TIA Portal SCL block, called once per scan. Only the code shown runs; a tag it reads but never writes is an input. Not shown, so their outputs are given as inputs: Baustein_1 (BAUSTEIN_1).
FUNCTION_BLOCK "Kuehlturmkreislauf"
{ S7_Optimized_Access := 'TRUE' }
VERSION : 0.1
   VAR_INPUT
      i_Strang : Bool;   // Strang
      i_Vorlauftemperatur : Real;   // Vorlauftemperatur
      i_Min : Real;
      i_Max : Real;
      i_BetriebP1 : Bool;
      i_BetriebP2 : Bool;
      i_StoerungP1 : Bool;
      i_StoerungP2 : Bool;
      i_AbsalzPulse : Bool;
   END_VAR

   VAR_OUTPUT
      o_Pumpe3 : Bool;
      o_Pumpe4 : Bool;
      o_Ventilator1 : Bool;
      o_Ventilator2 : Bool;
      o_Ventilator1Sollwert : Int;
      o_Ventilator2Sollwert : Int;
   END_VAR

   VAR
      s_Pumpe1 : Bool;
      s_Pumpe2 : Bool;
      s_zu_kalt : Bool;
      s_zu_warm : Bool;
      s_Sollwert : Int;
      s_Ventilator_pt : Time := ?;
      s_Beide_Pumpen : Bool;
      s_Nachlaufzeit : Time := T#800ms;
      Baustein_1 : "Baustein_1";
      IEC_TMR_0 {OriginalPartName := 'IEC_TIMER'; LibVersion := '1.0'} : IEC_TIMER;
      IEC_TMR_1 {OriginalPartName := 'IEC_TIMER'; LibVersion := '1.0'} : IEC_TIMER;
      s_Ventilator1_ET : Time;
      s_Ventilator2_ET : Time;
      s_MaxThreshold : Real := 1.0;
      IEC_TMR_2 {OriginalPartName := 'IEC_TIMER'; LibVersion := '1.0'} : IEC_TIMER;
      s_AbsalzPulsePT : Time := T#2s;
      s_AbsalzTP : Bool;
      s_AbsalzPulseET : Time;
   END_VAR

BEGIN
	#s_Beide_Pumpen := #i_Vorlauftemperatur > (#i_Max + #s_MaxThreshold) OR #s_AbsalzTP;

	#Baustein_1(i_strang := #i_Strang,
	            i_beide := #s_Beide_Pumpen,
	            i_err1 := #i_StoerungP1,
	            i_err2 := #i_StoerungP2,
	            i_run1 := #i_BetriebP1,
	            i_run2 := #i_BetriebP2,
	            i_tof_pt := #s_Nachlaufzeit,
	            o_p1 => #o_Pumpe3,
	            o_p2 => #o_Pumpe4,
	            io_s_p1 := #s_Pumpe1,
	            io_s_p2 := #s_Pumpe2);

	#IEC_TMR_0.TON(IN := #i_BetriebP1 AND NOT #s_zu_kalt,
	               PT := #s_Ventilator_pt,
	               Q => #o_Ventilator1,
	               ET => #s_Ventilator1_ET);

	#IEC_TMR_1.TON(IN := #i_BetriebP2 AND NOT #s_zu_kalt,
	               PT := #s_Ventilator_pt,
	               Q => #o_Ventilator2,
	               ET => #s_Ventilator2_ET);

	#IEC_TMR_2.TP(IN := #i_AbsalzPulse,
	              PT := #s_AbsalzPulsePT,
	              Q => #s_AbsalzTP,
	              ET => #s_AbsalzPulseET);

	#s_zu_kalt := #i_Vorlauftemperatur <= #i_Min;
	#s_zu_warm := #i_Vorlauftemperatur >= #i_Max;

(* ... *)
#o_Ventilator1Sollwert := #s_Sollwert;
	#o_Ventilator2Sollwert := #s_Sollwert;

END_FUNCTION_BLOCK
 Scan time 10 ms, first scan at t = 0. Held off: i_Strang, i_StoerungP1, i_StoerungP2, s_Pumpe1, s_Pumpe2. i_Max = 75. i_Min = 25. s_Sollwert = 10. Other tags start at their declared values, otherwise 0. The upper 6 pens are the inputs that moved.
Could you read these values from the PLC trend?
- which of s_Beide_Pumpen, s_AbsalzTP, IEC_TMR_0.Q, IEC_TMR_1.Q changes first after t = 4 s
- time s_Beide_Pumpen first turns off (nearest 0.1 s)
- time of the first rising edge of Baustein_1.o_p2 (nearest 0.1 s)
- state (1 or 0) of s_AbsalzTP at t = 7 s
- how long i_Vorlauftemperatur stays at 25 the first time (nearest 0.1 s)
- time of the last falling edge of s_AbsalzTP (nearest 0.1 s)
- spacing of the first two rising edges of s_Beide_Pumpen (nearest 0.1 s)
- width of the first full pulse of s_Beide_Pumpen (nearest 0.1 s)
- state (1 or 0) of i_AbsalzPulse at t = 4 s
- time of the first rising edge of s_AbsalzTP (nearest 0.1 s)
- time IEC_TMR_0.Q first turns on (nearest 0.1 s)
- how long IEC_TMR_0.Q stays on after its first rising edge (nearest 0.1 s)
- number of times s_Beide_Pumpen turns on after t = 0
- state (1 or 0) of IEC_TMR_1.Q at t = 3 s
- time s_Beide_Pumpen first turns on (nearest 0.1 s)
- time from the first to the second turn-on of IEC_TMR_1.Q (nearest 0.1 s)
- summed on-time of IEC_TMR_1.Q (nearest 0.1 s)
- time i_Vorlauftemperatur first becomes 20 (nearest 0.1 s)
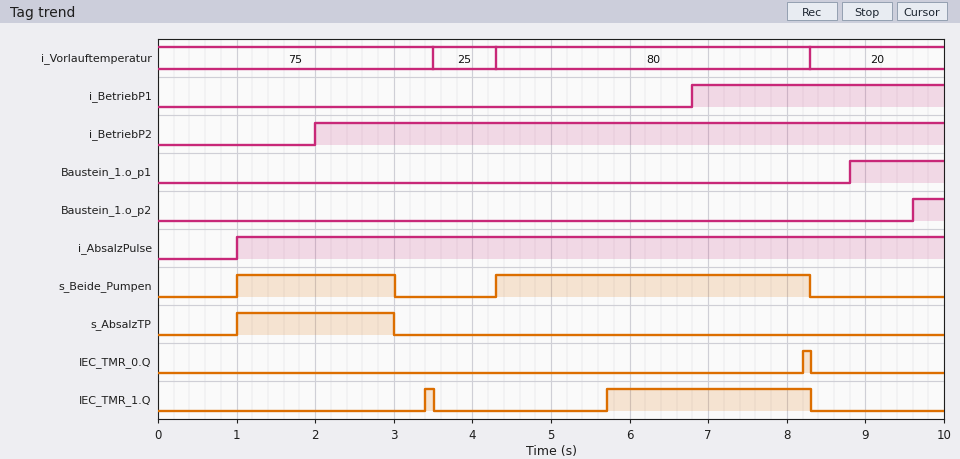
s_Beide_Pumpen
3.0 s
9.6 s
0
0.8 s
3.0 s
3.3 s
2.0 s
1
1.0 s
8.2 s
0.1 s
2
0
1.0 s
2.3 s
2.7 s
8.3 s
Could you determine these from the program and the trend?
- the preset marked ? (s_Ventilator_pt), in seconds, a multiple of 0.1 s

1.4 s
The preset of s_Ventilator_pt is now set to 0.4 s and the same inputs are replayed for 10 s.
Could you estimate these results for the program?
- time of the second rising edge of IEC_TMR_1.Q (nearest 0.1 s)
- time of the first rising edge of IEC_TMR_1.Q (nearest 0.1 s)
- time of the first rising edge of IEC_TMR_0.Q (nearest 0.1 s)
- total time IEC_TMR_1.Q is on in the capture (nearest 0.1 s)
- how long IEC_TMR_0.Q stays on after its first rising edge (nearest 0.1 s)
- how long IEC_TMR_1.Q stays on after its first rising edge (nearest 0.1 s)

4.7 s
2.4 s
7.2 s
4.7 s
1.1 s
1.1 s
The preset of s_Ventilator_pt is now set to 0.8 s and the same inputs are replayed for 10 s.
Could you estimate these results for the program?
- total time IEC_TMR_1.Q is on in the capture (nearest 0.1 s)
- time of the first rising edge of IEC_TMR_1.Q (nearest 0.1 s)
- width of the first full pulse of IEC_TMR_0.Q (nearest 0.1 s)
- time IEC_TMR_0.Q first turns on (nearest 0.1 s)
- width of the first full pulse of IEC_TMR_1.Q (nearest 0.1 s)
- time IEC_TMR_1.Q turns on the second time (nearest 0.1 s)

3.9 s
2.8 s
0.7 s
7.6 s
0.7 s
5.1 s
